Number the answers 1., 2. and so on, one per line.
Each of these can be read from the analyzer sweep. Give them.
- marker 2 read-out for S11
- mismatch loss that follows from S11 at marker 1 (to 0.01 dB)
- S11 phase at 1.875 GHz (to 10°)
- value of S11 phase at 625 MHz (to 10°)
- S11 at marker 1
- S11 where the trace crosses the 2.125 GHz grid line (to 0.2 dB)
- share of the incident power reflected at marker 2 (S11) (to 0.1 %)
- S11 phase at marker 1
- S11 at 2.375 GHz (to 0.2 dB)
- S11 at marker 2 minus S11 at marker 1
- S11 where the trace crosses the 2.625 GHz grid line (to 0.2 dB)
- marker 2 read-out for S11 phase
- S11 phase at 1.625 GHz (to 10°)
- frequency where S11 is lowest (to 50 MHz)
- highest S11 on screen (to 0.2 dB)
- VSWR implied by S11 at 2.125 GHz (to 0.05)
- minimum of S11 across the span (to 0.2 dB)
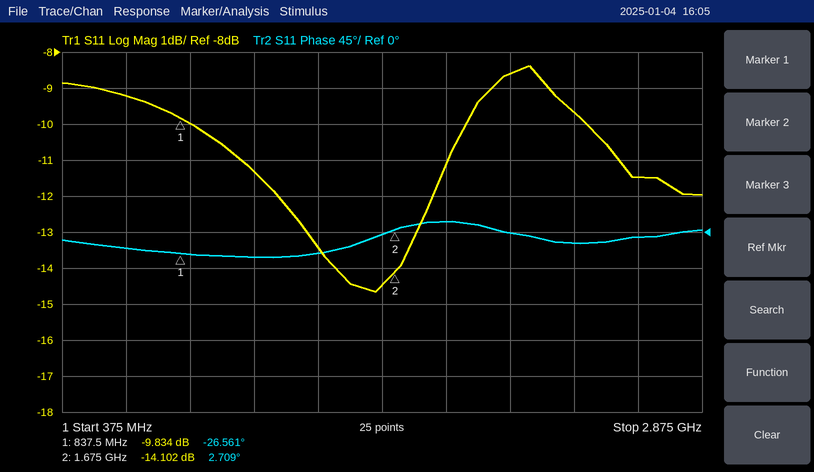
1. -14.102 dB
2. 0.48 dB
3. 10°
4. -20°
5. -9.834 dB
6. -8.6 dB
7. 3.9 %
8. -26.561°
9. -9.6 dB
10. -4.268 dB
11. -11.4 dB
12. 2.709°
13. 0°
14. 1.60 GHz
15. -8.4 dB
16. 2.20
17. -14.6 dB
